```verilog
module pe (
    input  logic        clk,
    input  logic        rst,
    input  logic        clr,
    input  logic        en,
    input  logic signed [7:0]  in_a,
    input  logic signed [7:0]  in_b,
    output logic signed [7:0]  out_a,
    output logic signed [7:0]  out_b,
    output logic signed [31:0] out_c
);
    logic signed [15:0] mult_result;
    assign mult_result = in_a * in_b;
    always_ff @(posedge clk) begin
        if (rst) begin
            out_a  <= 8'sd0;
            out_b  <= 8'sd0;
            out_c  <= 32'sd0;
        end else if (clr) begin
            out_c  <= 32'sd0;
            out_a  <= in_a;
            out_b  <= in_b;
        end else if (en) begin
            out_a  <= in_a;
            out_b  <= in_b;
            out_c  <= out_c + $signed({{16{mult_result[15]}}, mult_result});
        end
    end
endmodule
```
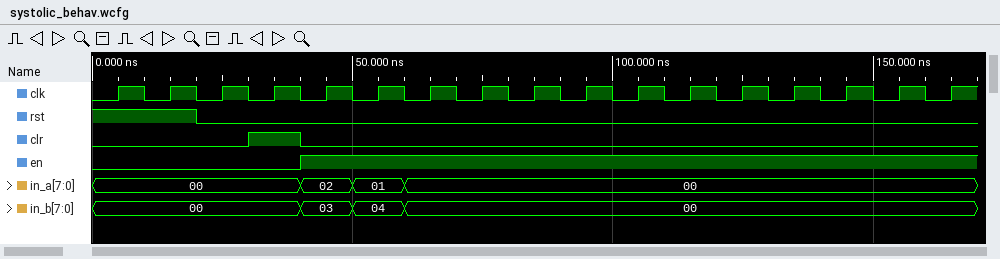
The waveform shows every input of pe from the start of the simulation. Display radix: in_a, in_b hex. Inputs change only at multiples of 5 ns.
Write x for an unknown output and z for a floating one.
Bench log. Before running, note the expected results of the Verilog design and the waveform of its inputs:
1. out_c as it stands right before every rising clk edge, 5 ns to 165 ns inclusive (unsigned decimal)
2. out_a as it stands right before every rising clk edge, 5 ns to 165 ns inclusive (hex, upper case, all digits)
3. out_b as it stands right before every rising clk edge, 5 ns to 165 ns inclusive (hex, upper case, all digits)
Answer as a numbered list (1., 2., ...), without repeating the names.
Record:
1. x, 0, 0, 0, 0, 6, 10, 10, 10, 10, 10, 10, 10, 10, 10, 10, 10
2. x, 00, 00, 00, 00, 02, 01, 00, 00, 00, 00, 00, 00, 00, 00, 00, 00
3. x, 00, 00, 00, 00, 03, 04, 00, 00, 00, 00, 00, 00, 00, 00, 00, 00
